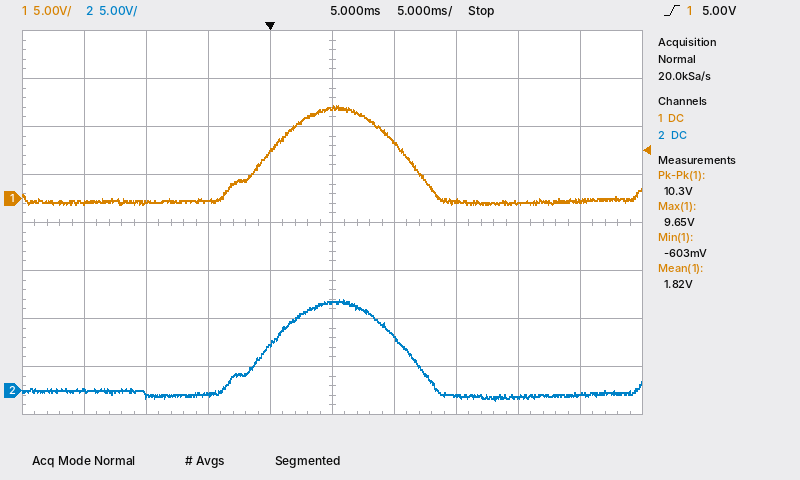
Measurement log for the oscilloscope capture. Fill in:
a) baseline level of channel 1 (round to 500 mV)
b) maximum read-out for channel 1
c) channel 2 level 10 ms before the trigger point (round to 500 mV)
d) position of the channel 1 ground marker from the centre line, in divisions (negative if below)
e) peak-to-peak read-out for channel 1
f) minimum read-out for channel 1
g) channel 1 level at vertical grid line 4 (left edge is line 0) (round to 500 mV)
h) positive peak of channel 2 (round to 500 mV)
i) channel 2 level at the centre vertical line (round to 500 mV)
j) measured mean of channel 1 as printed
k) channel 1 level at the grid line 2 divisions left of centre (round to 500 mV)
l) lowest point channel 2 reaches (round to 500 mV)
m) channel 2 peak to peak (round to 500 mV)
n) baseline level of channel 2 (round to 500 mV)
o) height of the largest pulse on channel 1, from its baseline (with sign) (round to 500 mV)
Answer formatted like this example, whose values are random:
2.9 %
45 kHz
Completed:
-500 mV
9.65 V
-500 mV
+0.5 div
10.3 V
-603 mV
5.0 V
9.5 V
9.0 V
1.82 V
0.0 V
-1.0 V
10.5 V
-500 mV
+10.0 V
